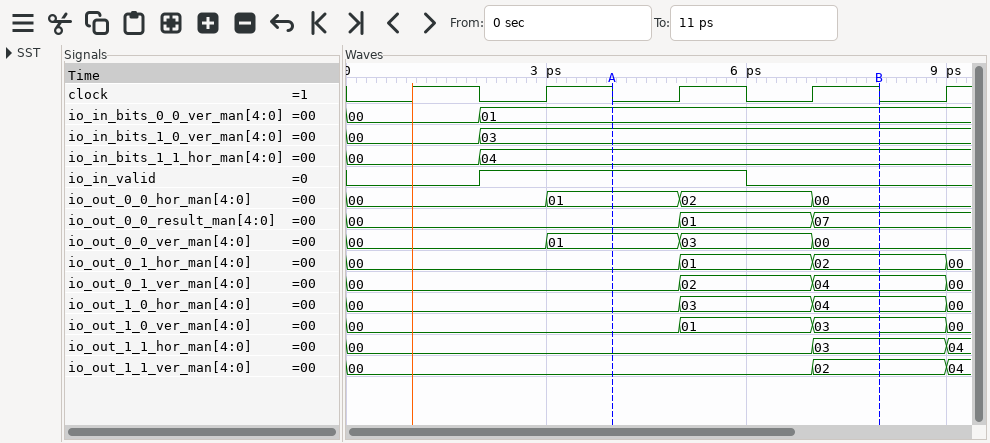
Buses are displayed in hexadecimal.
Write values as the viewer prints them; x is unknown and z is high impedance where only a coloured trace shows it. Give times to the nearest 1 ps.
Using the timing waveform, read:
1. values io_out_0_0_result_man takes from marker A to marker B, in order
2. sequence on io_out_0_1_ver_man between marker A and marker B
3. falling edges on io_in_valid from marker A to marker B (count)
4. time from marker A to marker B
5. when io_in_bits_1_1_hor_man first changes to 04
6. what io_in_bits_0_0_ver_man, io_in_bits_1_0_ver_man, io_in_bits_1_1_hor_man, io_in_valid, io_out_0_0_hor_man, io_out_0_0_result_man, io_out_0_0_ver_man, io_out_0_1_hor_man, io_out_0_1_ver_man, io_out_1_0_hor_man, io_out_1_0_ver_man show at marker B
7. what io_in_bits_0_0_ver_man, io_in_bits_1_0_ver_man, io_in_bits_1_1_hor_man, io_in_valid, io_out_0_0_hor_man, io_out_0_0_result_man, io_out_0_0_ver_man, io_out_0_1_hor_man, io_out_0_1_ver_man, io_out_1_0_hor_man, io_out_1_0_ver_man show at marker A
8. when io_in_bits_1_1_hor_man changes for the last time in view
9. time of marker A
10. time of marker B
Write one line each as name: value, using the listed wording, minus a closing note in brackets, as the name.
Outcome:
values io_out_0_0_result_man takes from marker A to marker B, in order: 00, 01, 07
sequence on io_out_0_1_ver_man between marker A and marker B: 00, 02, 04
falling edges on io_in_valid from marker A to marker B: 1
time from marker A to marker B: 4 ps
when io_in_bits_1_1_hor_man first changes to 04: 2 ps
what io_in_bits_0_0_ver_man, io_in_bits_1_0_ver_man, io_in_bits_1_1_hor_man, io_in_valid, io_out_0_0_hor_man, io_out_0_0_result_man, io_out_0_0_ver_man, io_out_0_1_hor_man, io_out_0_1_ver_man, io_out_1_0_hor_man, io_out_1_0_ver_man show at marker B: io_in_bits_0_0_ver_man=01, io_in_bits_1_0_ver_man=03, io_in_bits_1_1_hor_man=04, io_in_valid=0, io_out_0_0_hor_man=00, io_out_0_0_result_man=07, io_out_0_0_ver_man=00, io_out_0_1_hor_man=02, io_out_0_1_ver_man=04, io_out_1_0_hor_man=04, io_out_1_0_ver_man=03
what io_in_bits_0_0_ver_man, io_in_bits_1_0_ver_man, io_in_bits_1_1_hor_man, io_in_valid, io_out_0_0_hor_man, io_out_0_0_result_man, io_out_0_0_ver_man, io_out_0_1_hor_man, io_out_0_1_ver_man, io_out_1_0_hor_man, io_out_1_0_ver_man show at marker A: io_in_bits_0_0_ver_man=01, io_in_bits_1_0_ver_man=03, io_in_bits_1_1_hor_man=04, io_in_valid=1, io_out_0_0_hor_man=01, io_out_0_0_result_man=00, io_out_0_0_ver_man=01, io_out_0_1_hor_man=00, io_out_0_1_ver_man=00, io_out_1_0_hor_man=00, io_out_1_0_ver_man=00
when io_in_bits_1_1_hor_man changes for the last time in view: 2 ps
time of marker A: 4 ps
time of marker B: 8 ps
